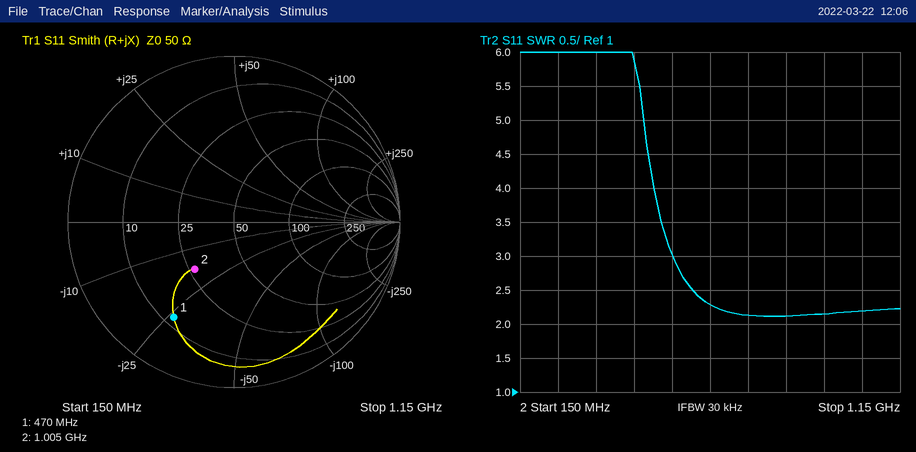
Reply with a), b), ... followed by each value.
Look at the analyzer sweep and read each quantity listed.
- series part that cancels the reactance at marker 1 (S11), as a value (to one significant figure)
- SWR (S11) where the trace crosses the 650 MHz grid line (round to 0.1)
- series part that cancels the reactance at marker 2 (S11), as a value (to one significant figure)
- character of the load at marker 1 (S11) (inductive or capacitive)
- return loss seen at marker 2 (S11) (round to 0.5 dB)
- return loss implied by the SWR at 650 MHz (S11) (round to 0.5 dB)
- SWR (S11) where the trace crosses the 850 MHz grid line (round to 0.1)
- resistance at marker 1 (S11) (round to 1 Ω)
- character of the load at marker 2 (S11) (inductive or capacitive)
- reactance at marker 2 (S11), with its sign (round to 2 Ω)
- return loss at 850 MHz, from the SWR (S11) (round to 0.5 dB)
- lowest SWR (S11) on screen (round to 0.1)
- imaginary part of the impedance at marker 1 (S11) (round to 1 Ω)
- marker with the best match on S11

a) 9 nH
b) 2.3
c) 3 nH
d) capacitive
e) 8.5 dB
f) 8.0 dB
g) 2.1
h) 12 Ω
i) capacitive
j) -18 Ω
k) 9.0 dB
l) 2.1
m) -26 Ω
n) marker 2
